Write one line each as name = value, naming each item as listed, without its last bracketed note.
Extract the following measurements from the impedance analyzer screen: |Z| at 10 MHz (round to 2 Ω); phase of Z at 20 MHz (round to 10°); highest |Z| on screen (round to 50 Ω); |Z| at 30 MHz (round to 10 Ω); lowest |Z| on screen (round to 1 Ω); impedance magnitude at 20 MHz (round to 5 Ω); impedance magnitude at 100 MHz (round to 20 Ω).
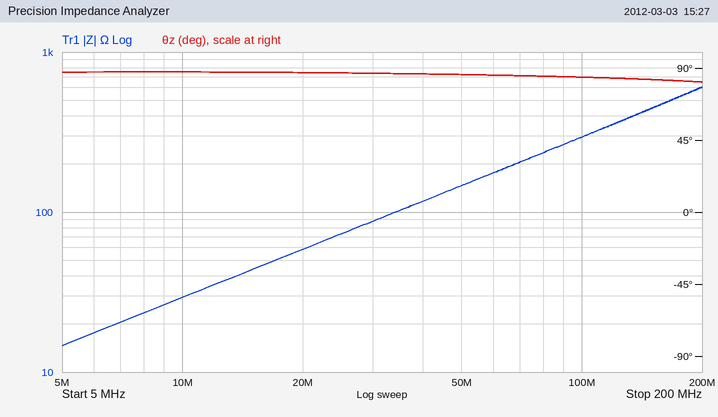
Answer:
|Z| at 10 MHz = 30 Ω
phase of Z at 20 MHz = 90°
highest |Z| on screen = 600 Ω
|Z| at 30 MHz = 90 Ω
lowest |Z| on screen = 15 Ω
impedance magnitude at 20 MHz = 60 Ω
impedance magnitude at 100 MHz = 300 Ω
